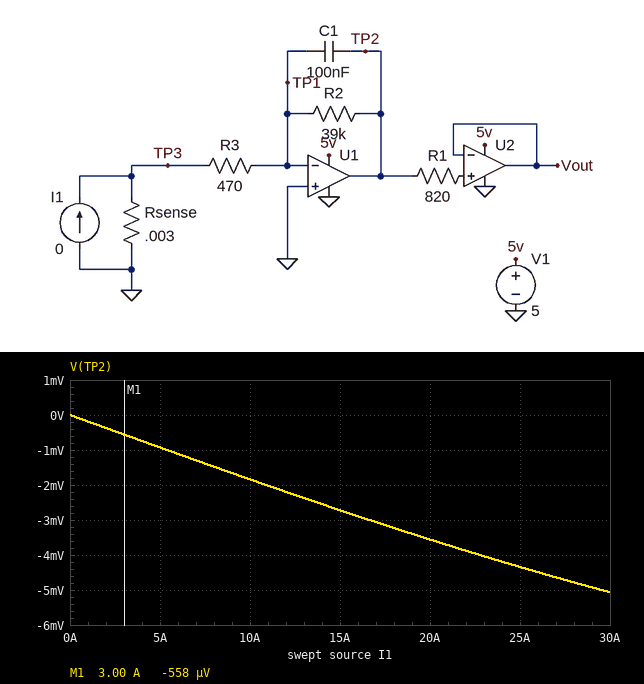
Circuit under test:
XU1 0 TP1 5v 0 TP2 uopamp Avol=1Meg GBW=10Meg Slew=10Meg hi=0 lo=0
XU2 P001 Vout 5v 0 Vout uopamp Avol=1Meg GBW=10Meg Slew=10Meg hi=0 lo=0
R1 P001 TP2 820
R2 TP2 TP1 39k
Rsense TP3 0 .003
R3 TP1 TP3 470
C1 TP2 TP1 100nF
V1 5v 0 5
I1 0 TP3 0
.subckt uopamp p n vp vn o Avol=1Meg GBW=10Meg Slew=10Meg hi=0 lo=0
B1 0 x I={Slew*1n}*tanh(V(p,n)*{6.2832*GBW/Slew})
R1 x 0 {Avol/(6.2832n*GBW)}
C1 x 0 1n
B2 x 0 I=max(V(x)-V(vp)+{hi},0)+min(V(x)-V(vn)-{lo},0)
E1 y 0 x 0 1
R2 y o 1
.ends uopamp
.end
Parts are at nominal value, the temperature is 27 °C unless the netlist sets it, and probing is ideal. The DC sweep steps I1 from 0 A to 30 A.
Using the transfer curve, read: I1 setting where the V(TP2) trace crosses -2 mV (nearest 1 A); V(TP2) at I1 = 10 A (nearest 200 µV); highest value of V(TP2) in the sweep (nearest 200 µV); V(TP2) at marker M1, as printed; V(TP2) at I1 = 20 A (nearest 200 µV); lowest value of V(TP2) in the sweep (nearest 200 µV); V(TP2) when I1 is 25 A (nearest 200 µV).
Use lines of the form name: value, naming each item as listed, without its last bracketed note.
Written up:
I1 setting where the V(TP2) trace crosses -2 mV: 11 A
V(TP2) at I1 = 10 A: -1.8 mV
highest value of V(TP2) in the sweep: 0 V
V(TP2) at marker M1, as printed: -558 µV
V(TP2) at I1 = 20 A: -3.6 mV
lowest value of V(TP2) in the sweep: -5.0 mV
V(TP2) when I1 is 25 A: -4.4 mV
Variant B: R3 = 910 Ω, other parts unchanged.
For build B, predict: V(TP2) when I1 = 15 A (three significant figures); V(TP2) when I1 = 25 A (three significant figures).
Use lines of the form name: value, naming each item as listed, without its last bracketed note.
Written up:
V(TP2) when I1 = 15 A: -2.69 mV
V(TP2) when I1 = 25 A: -4.30 mV
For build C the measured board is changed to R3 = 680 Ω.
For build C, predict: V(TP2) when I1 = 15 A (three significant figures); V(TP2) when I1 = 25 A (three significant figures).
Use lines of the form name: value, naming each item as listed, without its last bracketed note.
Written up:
V(TP2) when I1 = 15 A: -2.71 mV
V(TP2) when I1 = 25 A: -4.32 mV
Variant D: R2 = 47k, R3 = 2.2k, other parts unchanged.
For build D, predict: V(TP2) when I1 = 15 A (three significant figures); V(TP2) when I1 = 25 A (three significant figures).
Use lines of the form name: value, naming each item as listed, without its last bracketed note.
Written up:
V(TP2) when I1 = 15 A: -2.63 mV
V(TP2) when I1 = 25 A: -4.21 mV
